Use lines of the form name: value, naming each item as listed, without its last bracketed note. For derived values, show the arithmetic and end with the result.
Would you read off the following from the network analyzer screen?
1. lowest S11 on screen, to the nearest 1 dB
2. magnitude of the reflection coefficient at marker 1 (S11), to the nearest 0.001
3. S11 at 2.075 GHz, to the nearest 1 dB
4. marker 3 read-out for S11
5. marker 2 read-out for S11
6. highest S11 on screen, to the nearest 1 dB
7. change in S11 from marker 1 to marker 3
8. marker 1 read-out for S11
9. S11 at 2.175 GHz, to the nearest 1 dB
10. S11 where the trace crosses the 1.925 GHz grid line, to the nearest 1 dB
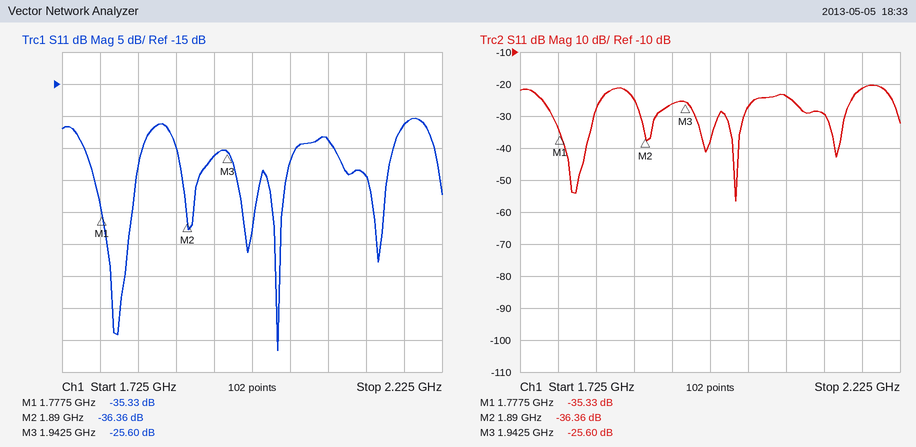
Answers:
lowest S11 on screen, to the nearest 1 dB: -57 dB
magnitude of the reflection coefficient at marker 1 (S11), to the nearest 0.001: 10^(-35.33/20) ≈ 0.017
S11 at 2.075 GHz, to the nearest 1 dB: -24 dB
marker 3 read-out for S11: -25.60 dB
marker 2 read-out for S11: -36.36 dB
highest S11 on screen, to the nearest 1 dB: -20 dB
change in S11 from marker 1 to marker 3: -25.6 − (-35.33) = 9.73 dB
marker 1 read-out for S11: -35.33 dB
S11 at 2.175 GHz, to the nearest 1 dB: -21 dB
S11 where the trace crosses the 1.925 GHz grid line, to the nearest 1 dB: -26 dB
